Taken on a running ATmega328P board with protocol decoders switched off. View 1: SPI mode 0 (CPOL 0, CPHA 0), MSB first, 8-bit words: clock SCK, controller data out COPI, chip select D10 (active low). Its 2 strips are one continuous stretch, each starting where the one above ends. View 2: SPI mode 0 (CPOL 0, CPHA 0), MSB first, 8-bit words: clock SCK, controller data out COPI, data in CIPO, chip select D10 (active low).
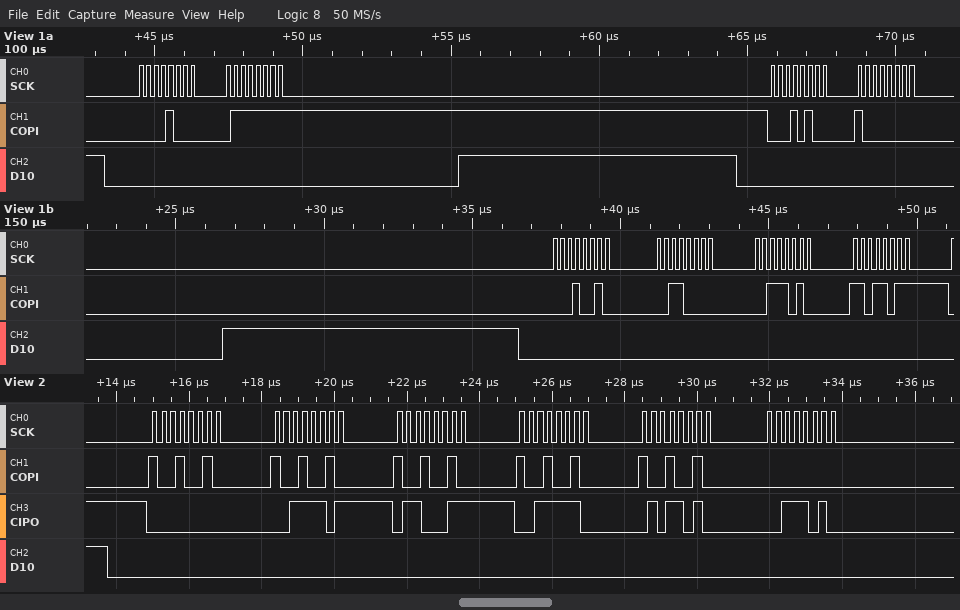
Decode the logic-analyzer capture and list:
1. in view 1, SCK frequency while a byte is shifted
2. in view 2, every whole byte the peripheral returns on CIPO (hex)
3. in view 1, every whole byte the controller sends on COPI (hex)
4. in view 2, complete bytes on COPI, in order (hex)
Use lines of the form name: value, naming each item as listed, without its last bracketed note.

in view 1, SCK frequency while a byte is shifted: 4 MHz
in view 2, every whole byte the peripheral returns on CIPO: 00 3D 63 3E 5A 3A
in view 1, every whole byte the controller sends on COPI: 08 7F 14 80 12 30 3A DB
in view 2, complete bytes on COPI, in order: 92 92 92 92 92 00
